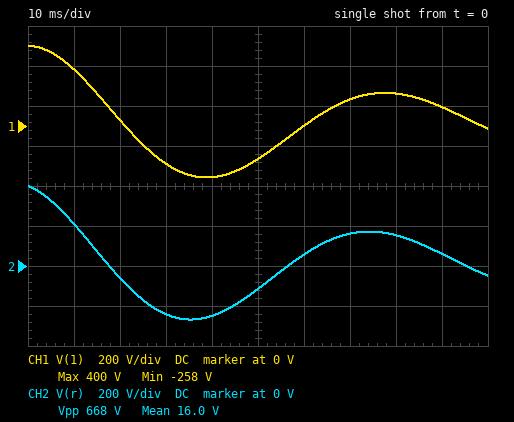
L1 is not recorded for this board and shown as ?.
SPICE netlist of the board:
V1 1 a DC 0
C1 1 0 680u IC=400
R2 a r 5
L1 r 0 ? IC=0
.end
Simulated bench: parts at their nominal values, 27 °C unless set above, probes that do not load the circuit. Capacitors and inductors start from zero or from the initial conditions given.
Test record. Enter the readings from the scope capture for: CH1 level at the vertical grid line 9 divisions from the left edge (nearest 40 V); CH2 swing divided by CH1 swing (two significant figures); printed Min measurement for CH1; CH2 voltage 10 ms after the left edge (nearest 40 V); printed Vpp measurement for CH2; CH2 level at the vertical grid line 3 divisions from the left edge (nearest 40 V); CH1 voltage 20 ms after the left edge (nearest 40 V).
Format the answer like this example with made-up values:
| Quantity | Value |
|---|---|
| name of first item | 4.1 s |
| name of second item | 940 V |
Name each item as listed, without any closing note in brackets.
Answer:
| Quantity | Value |
|---|---|
| CH1 level at the vertical grid line 9 divisions from the left edge | 80 V |
| CH2 swing divided by CH1 swing | 1.0 |
| printed Min measurement for CH1 | -258 V |
| CH2 voltage 10 ms after the left edge | 200 V |
| printed Vpp measurement for CH2 | 668 V |
| CH2 level at the vertical grid line 3 divisions from the left edge | -240 V |
| CH1 voltage 20 ms after the left edge | 40 V |
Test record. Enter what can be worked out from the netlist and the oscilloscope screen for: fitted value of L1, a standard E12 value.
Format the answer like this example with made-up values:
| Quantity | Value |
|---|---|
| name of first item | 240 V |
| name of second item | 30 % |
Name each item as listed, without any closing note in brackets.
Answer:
| Quantity | Value |
|---|---|
| fitted value of L1, a standard E12 value | 220 mH |
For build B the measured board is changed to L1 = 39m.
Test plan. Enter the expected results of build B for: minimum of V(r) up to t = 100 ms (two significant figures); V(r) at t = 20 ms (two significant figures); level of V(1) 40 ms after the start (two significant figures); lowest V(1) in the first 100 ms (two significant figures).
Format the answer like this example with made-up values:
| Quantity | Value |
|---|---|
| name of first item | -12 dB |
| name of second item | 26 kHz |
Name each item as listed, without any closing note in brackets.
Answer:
| Quantity | Value |
|---|---|
| minimum of V(r) up to t = 100 ms | -170 V |
| V(r) at t = 20 ms | -77 V |
| level of V(1) 40 ms after the start | 25 V |
| lowest V(1) in the first 100 ms | -130 V |
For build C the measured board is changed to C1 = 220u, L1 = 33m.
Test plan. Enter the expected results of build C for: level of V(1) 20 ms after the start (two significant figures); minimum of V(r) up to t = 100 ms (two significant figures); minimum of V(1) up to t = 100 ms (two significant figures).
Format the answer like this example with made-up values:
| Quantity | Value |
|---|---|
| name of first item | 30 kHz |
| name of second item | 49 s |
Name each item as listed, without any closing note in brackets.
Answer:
| Quantity | Value |
|---|---|
| level of V(1) 20 ms after the start | 64 V |
| minimum of V(r) up to t = 100 ms | -230 V |
| minimum of V(1) up to t = 100 ms | -210 V |
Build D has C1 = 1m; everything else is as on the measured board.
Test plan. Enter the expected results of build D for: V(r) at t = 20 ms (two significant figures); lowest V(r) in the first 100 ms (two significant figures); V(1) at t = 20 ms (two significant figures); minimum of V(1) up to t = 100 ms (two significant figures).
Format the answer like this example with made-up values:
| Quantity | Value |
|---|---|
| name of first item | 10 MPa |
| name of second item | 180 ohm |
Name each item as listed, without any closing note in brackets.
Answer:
| Quantity | Value |
|---|---|
| V(r) at t = 20 ms | 23 V |
| lowest V(r) in the first 100 ms | -250 V |
| V(1) at t = 20 ms | 130 V |
| minimum of V(1) up to t = 100 ms | -230 V |
